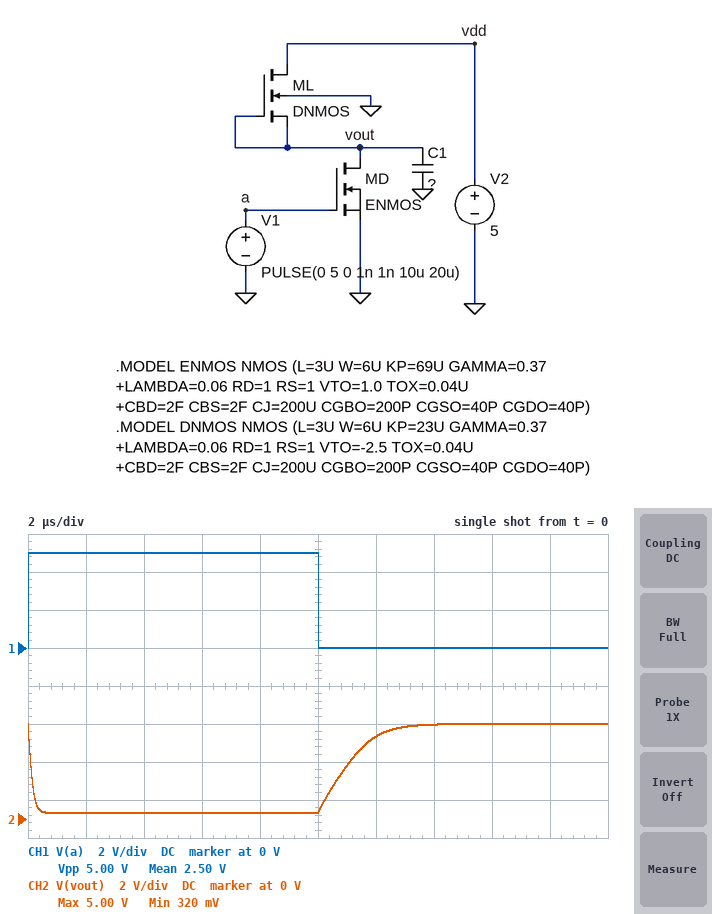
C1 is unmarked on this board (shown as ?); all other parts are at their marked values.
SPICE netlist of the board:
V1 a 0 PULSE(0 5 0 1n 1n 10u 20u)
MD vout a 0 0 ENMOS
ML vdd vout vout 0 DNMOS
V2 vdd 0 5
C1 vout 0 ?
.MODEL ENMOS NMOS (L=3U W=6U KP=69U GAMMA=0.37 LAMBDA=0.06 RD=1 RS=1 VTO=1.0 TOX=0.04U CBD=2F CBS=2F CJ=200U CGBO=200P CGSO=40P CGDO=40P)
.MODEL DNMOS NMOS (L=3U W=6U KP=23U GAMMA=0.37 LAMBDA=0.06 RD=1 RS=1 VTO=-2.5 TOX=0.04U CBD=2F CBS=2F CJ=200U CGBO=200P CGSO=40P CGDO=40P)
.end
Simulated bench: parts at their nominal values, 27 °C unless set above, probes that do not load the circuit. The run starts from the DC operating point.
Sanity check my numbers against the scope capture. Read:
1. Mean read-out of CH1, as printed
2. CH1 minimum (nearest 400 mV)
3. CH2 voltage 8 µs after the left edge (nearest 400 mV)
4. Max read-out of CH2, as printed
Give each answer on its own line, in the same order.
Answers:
2.50 V
0 V
400 mV
5.00 V
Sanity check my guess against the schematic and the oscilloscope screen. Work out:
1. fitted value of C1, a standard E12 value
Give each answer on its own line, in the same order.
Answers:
56 pF
